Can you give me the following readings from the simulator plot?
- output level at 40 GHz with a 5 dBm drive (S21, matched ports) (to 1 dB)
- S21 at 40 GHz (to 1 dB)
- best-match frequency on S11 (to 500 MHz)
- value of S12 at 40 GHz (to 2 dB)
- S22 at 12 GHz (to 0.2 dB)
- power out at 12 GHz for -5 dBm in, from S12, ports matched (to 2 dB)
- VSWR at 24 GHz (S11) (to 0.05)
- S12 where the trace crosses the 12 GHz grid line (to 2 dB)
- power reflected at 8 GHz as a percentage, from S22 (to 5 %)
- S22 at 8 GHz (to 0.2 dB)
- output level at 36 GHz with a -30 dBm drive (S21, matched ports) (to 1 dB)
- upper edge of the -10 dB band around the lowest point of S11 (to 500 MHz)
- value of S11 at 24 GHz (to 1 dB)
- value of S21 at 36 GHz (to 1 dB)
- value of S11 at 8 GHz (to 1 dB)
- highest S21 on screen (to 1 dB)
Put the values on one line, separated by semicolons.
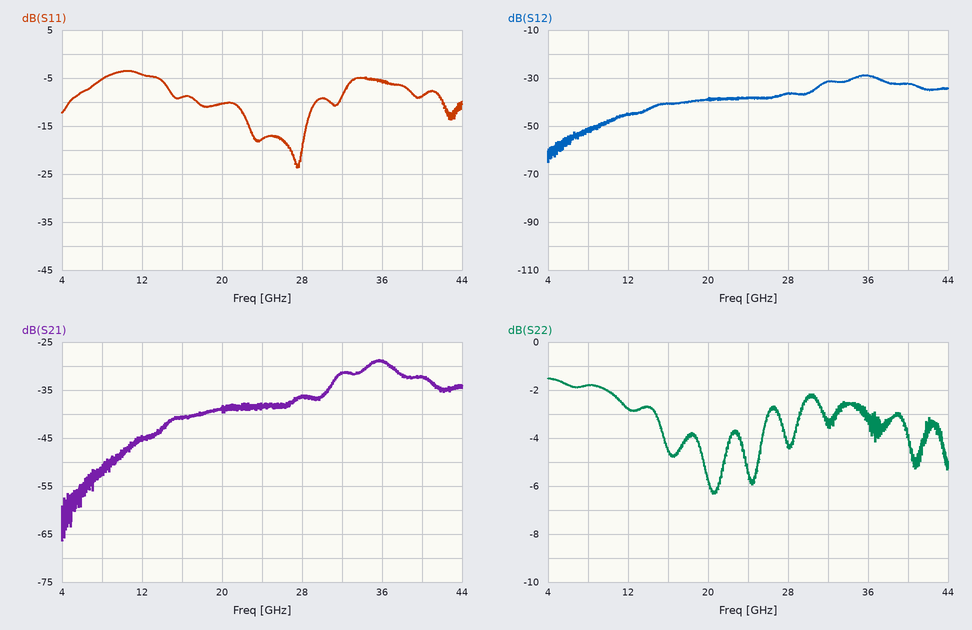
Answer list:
-27 dBm; -32 dB; 27.5 GHz; -32 dB; -2.8 dB; -50 dBm; 1.30; -46 dB; 65 %; -1.8 dB; -59 dBm; 29.5 GHz; -18 dB; -29 dB; -5 dB; -29 dB
